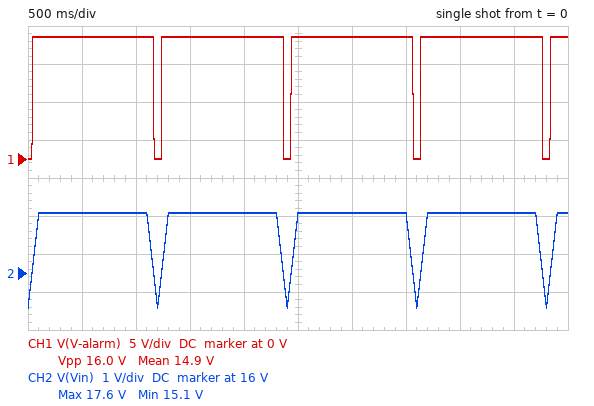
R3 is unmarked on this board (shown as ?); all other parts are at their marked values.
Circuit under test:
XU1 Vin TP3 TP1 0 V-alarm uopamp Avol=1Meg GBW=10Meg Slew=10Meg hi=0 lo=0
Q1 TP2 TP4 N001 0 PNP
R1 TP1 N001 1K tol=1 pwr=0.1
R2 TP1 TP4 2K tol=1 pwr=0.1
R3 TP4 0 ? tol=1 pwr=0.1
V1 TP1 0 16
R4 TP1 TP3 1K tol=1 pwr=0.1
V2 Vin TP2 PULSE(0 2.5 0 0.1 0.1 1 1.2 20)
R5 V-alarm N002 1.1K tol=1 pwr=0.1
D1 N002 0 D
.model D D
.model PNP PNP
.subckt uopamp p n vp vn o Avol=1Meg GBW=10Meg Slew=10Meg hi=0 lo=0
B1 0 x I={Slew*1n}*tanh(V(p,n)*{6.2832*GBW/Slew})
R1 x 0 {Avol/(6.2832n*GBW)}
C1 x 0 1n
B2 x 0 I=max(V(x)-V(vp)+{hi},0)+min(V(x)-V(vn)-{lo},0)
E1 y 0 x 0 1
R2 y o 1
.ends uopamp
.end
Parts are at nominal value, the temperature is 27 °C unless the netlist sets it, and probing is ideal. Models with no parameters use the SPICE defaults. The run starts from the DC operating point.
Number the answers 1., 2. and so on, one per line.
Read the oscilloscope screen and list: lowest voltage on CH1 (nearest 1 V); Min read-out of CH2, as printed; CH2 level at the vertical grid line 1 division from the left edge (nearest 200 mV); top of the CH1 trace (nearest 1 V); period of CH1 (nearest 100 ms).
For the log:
1. 0 V
2. 15.1 V
3. 17.6 V
4. 16 V
5. 1.2 s
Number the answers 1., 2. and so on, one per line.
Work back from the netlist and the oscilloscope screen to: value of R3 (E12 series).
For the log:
1. 8.2 kΩ
